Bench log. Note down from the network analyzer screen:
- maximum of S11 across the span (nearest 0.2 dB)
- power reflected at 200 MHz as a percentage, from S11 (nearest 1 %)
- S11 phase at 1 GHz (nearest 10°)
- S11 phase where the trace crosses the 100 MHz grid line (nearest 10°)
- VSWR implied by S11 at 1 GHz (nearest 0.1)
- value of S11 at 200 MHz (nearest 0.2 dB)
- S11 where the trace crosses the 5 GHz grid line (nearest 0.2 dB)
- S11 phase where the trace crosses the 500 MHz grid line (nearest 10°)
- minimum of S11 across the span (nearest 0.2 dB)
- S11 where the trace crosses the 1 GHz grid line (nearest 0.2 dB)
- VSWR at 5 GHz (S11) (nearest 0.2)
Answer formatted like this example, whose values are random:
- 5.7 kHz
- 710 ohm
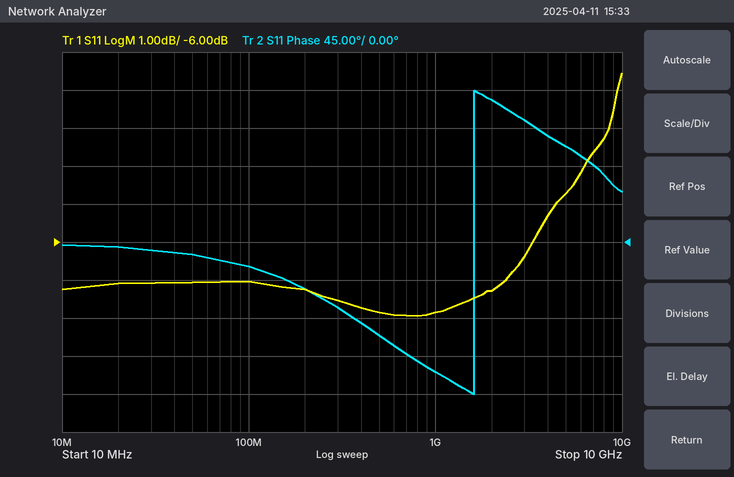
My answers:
- -1.6 dB
- 19 %
- -150°
- -30°
- 2.4
- -7.2 dB
- -4.8 dB
- -110°
- -8.0 dB
- -7.8 dB
- 3.8
